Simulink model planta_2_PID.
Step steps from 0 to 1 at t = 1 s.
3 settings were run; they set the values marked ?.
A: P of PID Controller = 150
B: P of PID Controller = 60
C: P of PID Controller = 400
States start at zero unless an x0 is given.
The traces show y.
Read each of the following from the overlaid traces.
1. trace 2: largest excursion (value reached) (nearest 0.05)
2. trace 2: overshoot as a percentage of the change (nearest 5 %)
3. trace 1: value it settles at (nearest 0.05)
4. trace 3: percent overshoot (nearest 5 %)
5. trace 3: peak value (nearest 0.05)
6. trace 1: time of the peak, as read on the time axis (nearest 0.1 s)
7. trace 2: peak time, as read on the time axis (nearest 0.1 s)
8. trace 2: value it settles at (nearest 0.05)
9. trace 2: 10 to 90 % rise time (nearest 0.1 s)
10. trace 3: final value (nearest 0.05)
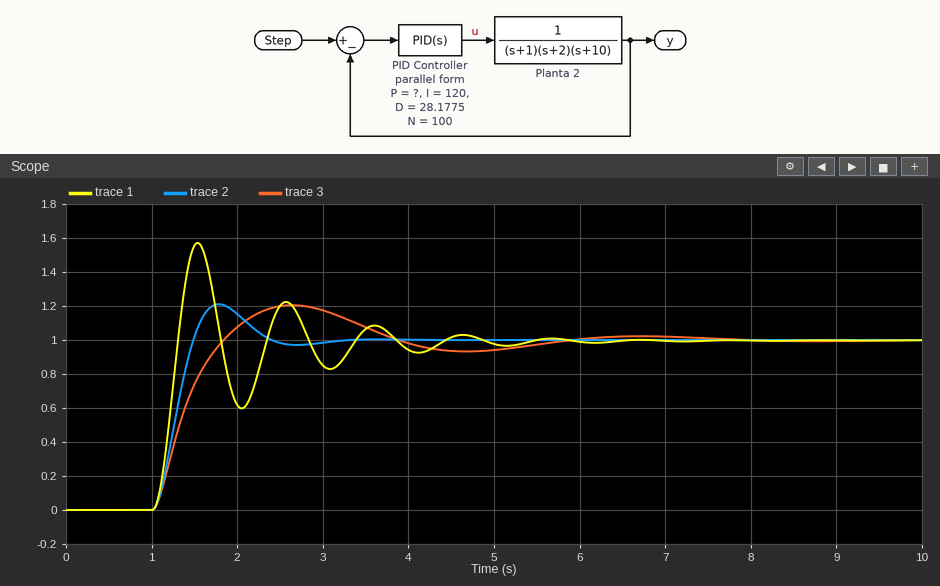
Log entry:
1.20
20 %
1.00
20 %
1.20
1.5 s
1.8 s
1.00
0.3 s
1.00
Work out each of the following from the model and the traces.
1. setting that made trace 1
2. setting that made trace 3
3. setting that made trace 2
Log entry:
C
B
A
